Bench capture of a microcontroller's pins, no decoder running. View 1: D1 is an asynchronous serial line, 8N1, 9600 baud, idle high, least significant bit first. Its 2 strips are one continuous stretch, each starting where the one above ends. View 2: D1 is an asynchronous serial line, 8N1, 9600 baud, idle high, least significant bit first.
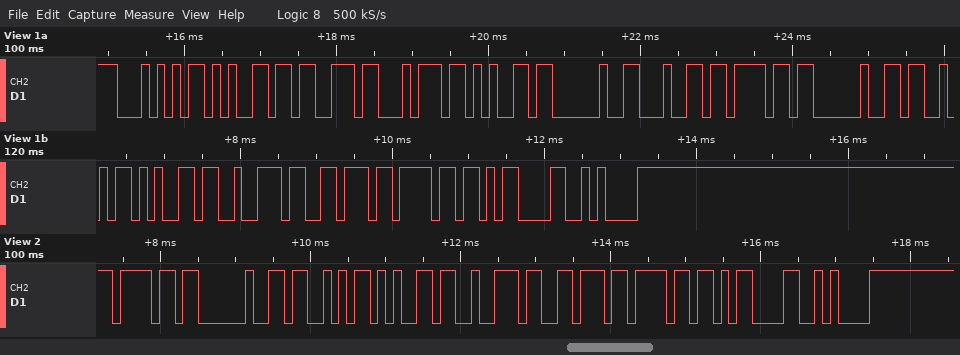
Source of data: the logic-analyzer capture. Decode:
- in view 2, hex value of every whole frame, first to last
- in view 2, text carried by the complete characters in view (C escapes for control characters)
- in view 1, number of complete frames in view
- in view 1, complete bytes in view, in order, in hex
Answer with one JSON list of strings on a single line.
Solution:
["6F 20 53 65 72 76 6F 0D 0A", "\"o Servo\\r\\n\"", "16", "54 65 73 74 65 20 64 6F 20 53 65 72 76 6F 0D 0A"]
